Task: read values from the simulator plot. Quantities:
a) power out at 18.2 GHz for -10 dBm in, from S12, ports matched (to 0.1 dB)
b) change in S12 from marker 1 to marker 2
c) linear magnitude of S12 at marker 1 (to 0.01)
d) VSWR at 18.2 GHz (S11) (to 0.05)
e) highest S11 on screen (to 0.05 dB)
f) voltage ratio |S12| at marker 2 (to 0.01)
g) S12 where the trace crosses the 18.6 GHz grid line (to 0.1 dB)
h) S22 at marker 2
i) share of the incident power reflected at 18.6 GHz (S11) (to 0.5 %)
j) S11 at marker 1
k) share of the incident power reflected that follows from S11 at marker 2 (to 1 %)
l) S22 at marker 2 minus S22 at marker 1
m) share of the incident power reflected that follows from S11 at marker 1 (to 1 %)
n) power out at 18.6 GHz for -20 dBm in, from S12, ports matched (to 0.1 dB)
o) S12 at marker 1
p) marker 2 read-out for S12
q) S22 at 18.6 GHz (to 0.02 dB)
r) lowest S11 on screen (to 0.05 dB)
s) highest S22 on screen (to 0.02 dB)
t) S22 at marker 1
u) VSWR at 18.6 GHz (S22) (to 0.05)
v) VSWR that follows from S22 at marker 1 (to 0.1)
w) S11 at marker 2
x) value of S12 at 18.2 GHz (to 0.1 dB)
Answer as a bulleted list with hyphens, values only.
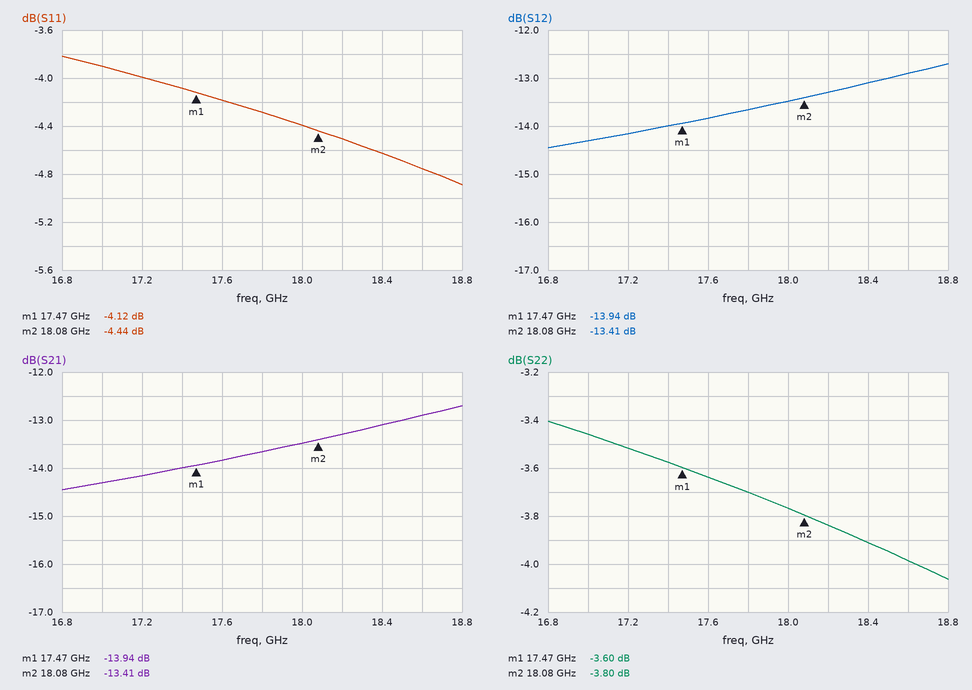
- -23.3 dBm
- 0.53 dB
- 0.20
- 3.95
- -3.80 dB
- 0.21
- -12.9 dB
- -3.80 dB
- 33.5 %
- -4.12 dB
- 36 %
- -0.20 dB
- 39 %
- -32.9 dBm
- -13.94 dB
- -13.41 dB
- -3.98 dB
- -4.90 dB
- -3.40 dB
- -3.60 dB
- 4.45
- 4.9
- -4.44 dB
- -13.3 dB
